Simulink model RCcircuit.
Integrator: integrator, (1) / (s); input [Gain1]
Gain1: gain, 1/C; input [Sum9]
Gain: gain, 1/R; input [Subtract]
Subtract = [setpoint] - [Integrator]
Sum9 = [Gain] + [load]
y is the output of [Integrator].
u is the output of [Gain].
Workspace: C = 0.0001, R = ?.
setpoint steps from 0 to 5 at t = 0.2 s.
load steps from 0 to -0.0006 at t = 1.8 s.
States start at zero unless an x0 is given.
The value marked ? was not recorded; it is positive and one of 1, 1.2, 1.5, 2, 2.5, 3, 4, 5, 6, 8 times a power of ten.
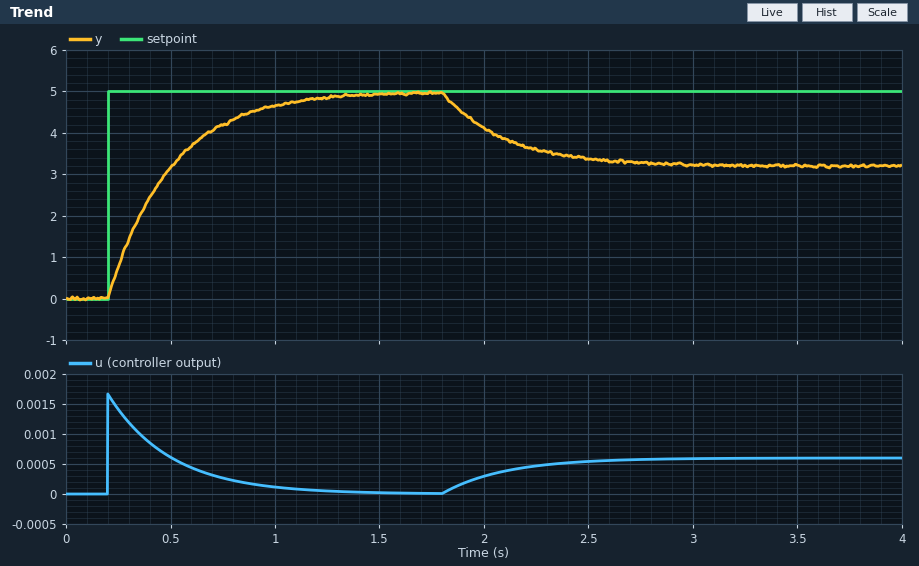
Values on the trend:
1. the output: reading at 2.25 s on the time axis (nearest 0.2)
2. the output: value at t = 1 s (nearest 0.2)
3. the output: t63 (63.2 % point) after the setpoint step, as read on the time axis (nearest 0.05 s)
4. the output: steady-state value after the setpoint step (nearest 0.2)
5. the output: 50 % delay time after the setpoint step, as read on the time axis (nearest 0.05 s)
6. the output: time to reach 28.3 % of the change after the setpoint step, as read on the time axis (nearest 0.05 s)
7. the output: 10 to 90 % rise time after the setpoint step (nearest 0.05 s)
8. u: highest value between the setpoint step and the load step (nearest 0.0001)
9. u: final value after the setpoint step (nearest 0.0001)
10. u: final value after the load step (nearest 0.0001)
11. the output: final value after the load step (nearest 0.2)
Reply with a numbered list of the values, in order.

1. 3.6
2. 4.6
3. 0.50 s
4. 5.0
5. 0.40 s
6. 0.30 s
7. 0.65 s
8. 0.0017
9. 0.0000
10. 0.0006
11. 3.2
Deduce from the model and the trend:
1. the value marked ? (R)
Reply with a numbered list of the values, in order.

1. 3000
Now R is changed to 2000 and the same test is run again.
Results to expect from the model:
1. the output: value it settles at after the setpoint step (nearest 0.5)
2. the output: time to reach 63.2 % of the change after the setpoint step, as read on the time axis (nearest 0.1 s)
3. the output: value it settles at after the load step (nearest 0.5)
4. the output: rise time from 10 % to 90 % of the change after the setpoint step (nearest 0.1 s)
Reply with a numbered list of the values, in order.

1. 5.0
2. 0.4 s
3. 4.0
4. 0.4 s
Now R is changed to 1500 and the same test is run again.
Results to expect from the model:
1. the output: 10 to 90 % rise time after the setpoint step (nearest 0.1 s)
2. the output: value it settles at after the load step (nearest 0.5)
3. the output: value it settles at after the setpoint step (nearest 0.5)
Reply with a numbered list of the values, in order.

1. 0.3 s
2. 4.0
3. 5.0
